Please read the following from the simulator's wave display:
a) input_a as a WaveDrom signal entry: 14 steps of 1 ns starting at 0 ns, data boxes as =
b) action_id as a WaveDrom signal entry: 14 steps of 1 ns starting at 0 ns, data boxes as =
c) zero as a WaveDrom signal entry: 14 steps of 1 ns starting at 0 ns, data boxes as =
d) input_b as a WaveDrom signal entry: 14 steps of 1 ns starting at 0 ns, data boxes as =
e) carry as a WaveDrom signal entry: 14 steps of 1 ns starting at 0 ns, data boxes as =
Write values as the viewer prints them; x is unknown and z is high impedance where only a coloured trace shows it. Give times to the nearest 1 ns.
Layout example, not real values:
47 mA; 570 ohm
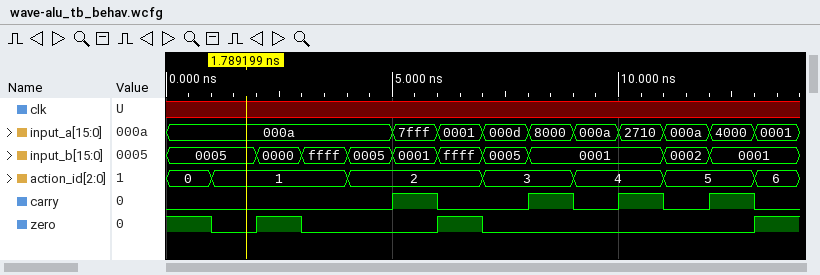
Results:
{name: 'input_a', wave: '=....=========', data: '000a 7fff 0001 000d 8000 000a 2710 000a 4000 0001'}; {name: 'action_id', wave: '==..=..=.=.=.=', data: '0 1 2 3 4 5 6'}; {name: 'zero', wave: '1010..10.....1'}; {name: 'input_b', wave: '=.=======..==.', data: '0005 0000 ffff 0005 0001 ffff 0005 0001 0002 0001'}; {name: 'carry', wave: '0....10.101010'}
